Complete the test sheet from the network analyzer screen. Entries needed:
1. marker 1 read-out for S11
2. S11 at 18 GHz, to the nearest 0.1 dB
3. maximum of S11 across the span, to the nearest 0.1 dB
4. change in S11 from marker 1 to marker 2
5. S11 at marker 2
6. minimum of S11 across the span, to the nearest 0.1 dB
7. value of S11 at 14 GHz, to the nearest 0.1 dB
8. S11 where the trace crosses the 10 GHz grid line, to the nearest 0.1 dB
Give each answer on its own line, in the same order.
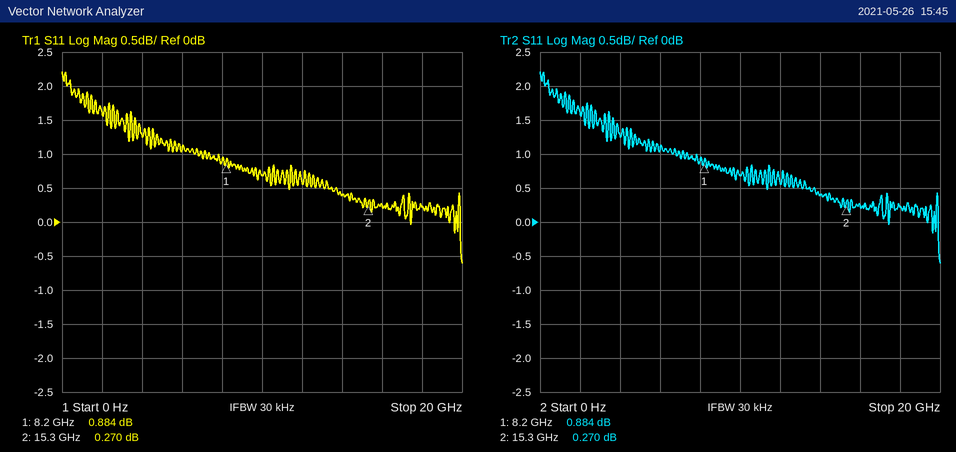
0.884 dB
0.2 dB
2.2 dB
-0.614 dB
0.270 dB
-0.6 dB
0.4 dB
0.7 dB
